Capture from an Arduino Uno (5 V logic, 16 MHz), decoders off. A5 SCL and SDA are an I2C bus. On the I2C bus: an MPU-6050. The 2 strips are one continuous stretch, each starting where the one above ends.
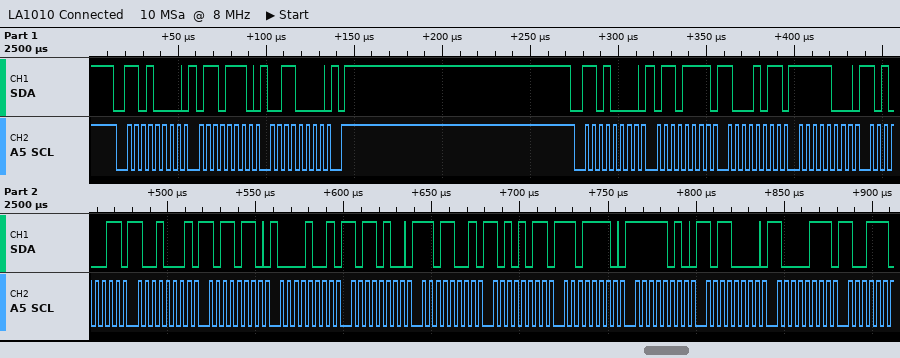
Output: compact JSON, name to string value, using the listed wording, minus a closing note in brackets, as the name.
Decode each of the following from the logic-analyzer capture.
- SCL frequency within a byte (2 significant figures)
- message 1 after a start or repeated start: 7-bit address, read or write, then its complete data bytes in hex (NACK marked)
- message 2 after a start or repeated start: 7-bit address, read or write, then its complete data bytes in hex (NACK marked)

{"SCL frequency within a byte": "250 kHz", "message 1 after a start or repeated start: 7-bit address, read or write, then its complete data bytes in hex": "0x68 write: 6E 30", "message 2 after a start or repeated start: 7-bit address, read or write, then its complete data bytes in hex": "0x68 write: 6F 8B F8 A3 91 B6 09 B4 D9 AB DE FA B0 87"}
